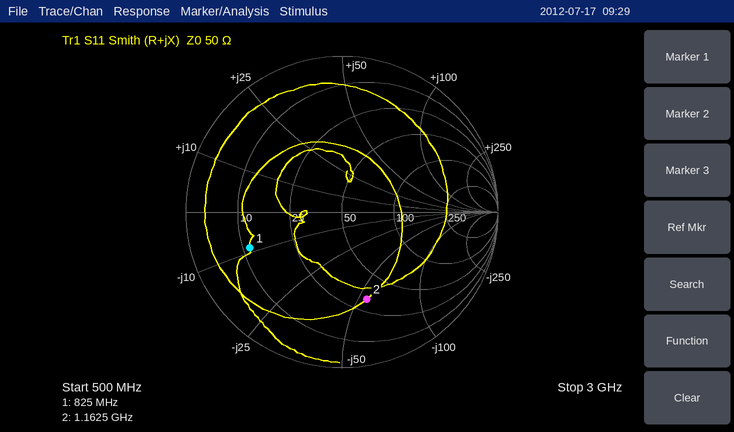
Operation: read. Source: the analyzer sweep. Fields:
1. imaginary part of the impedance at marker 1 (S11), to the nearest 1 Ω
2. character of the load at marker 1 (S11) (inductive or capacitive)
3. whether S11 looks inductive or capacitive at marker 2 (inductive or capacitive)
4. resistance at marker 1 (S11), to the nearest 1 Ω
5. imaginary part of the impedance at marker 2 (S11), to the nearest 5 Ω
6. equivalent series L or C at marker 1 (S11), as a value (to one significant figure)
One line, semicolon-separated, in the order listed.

-9 Ω; capacitive; capacitive; 12 Ω; -55 Ω; 20 pF
